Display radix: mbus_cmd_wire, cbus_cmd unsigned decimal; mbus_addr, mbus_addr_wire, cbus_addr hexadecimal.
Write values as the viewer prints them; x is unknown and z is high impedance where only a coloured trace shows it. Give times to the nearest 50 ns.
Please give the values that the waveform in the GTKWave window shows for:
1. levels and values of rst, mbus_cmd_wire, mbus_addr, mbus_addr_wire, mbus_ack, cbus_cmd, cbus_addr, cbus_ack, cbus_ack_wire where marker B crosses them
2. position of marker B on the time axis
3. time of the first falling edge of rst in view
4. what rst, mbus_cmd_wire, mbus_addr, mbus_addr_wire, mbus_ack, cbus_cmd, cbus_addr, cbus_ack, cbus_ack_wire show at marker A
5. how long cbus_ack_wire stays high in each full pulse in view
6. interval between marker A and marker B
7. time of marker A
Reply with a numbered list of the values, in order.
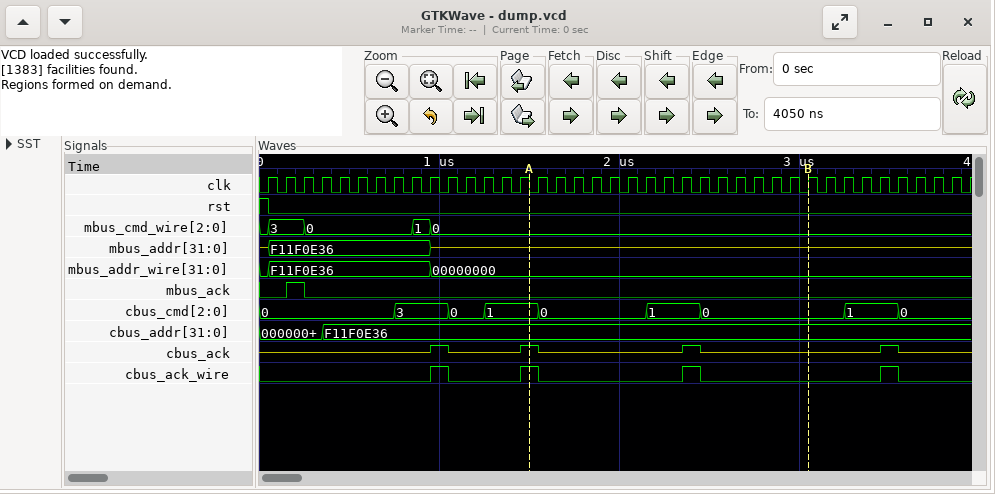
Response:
1. rst=0, mbus_cmd_wire=0, mbus_addr=z, mbus_addr_wire=00000000, mbus_ack=0, cbus_cmd=0, cbus_addr=F11F0E36, cbus_ack=z, cbus_ack_wire=0
2. 3050 ns
3. 50 ns
4. rst=0, mbus_cmd_wire=0, mbus_addr=z, mbus_addr_wire=00000000, mbus_ack=0, cbus_cmd=1, cbus_addr=F11F0E36, cbus_ack=1, cbus_ack_wire=1
5. 100 ns, 100 ns, 100 ns, 100 ns
6. 1550 ns
7. 1500 ns
